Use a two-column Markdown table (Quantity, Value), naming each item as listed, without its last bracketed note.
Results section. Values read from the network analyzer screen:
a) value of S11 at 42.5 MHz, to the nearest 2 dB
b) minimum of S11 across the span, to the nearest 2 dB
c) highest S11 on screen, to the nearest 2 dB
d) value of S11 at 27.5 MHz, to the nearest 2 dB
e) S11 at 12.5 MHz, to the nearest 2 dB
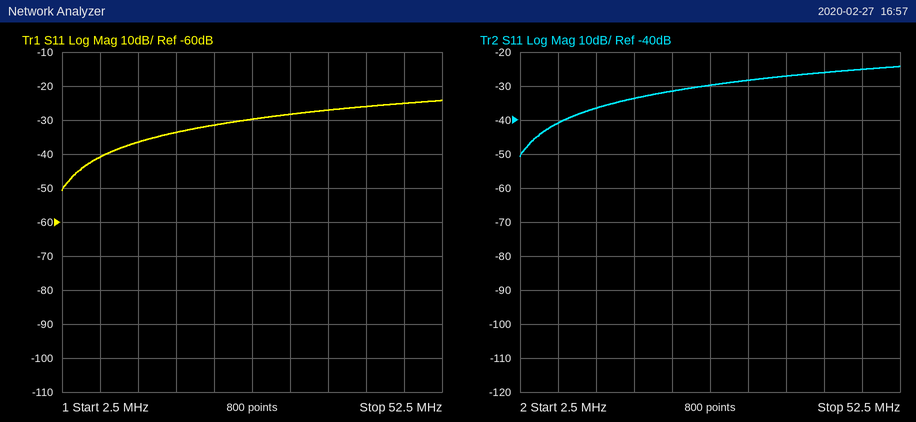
| Quantity | Value |
|---|---|
| value of S11 at 42.5 MHz, to the nearest 2 dB | -26 dB |
| minimum of S11 across the span, to the nearest 2 dB | -50 dB |
| highest S11 on screen, to the nearest 2 dB | -24 dB |
| value of S11 at 27.5 MHz, to the nearest 2 dB | -30 dB |
| S11 at 12.5 MHz, to the nearest 2 dB | -36 dB |
